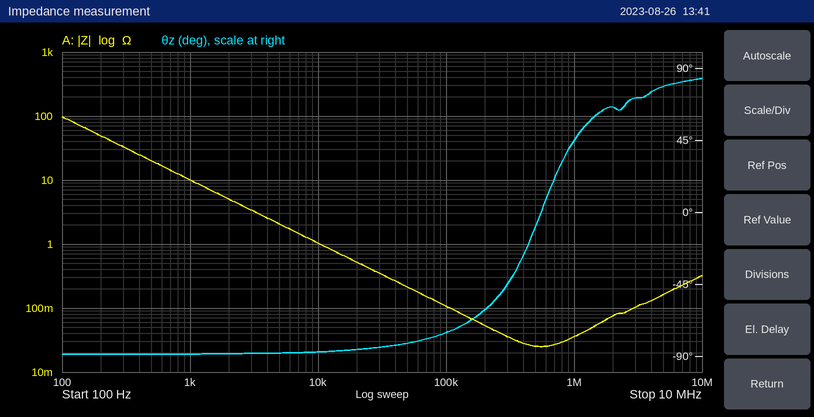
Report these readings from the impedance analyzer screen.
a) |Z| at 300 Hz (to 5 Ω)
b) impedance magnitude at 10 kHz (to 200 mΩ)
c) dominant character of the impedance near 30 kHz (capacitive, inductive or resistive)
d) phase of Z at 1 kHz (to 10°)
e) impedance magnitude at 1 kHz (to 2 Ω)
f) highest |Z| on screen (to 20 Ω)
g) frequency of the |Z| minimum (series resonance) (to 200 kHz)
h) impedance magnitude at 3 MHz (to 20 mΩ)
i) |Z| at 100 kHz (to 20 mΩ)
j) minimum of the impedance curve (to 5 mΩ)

35 Ω
1.0 Ω
capacitive
-90°
10 Ω
100 Ω
600 kHz
100 mΩ
100 mΩ
25 mΩ
